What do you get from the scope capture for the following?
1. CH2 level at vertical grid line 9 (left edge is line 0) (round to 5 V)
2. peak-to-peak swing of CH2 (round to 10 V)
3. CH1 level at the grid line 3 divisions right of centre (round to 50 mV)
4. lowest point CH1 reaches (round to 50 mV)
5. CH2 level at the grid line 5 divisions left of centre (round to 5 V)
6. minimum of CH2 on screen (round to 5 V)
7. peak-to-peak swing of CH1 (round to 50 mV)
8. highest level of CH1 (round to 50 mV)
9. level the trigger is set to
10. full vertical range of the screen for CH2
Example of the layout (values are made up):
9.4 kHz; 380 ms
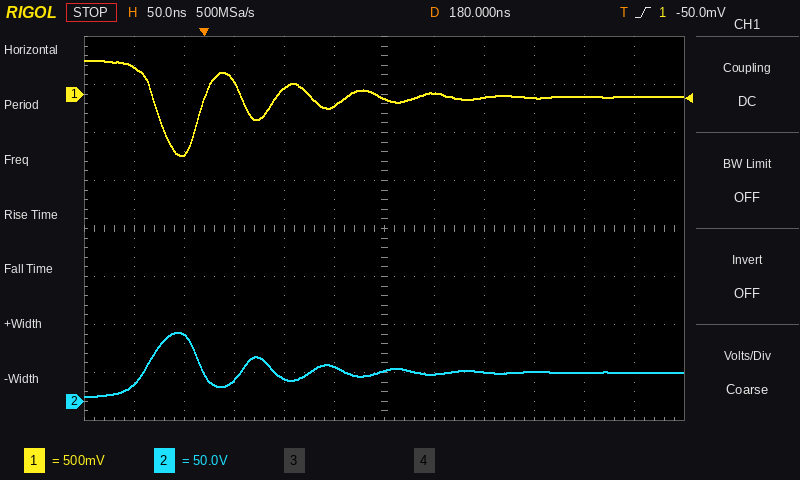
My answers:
30 V; 70 V; -50 mV; -650 mV; 20 V; 5 V; 1.00 V; 350 mV; -50.0 mV; 400 V
